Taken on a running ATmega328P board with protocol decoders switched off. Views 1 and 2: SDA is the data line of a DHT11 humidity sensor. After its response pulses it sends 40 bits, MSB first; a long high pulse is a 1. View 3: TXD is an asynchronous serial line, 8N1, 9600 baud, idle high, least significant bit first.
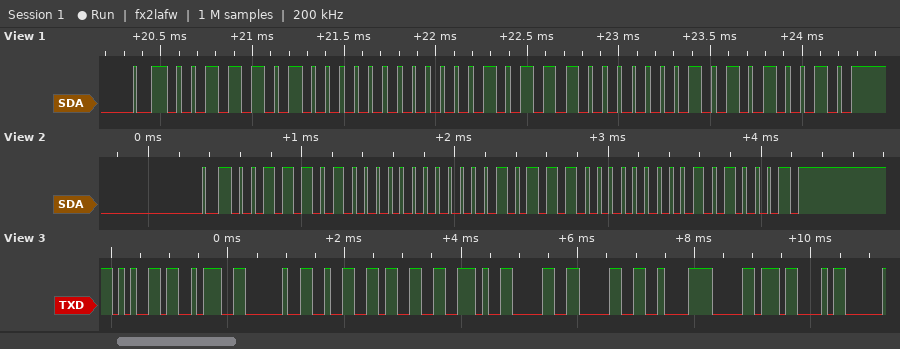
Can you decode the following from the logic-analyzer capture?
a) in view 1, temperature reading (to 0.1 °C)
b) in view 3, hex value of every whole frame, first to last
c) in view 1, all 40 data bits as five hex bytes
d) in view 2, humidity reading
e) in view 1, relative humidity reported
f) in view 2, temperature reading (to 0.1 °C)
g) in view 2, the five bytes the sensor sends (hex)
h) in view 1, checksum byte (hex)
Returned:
23.1 °C
65 3A 20 32 33 2E 30 30 C2 B0 43
3A 00 17 01 52
58 %
58 %
23.0 °C
3A 00 17 00 51
0x52
